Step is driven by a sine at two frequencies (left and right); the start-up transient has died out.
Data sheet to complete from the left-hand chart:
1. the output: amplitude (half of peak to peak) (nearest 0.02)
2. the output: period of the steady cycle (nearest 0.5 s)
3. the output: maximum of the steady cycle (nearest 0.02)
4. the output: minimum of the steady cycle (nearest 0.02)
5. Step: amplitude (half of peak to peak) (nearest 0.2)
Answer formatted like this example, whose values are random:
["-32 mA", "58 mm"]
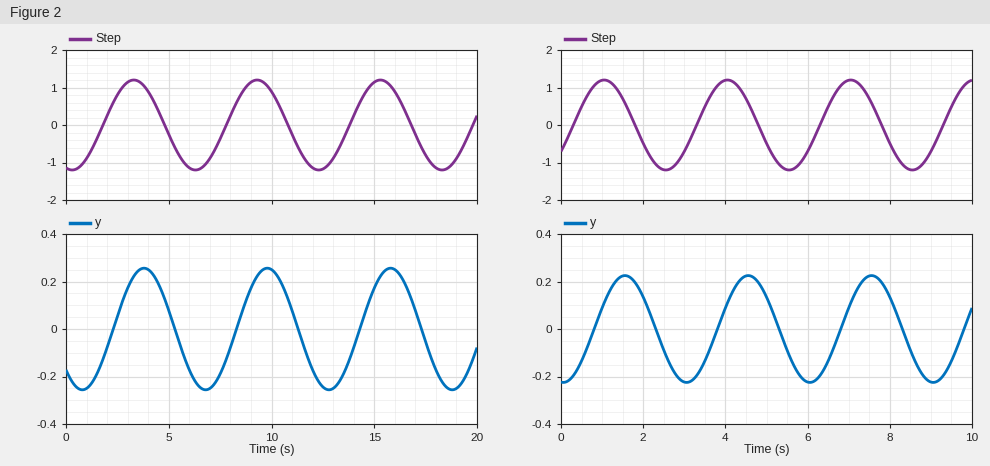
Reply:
["0.26", "6.0 s", "0.26", "-0.26", "1.2"]
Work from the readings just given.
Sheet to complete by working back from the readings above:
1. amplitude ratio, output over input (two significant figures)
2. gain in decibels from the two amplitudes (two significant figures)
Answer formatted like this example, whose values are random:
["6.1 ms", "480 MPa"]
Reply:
["0.22", "-13 dB"]
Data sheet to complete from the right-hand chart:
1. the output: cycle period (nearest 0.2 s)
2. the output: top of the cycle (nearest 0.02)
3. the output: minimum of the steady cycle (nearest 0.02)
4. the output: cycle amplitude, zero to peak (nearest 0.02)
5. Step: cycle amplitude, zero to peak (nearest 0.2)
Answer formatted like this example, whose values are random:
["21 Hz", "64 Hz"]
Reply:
["3.0 s", "0.22", "-0.22", "0.22", "1.2"]
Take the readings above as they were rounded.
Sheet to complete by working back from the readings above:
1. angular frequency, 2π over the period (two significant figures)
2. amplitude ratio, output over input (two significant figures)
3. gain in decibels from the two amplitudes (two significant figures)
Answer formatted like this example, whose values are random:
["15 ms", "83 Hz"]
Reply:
["2.1 rad/s", "0.18", "-15 dB"]
